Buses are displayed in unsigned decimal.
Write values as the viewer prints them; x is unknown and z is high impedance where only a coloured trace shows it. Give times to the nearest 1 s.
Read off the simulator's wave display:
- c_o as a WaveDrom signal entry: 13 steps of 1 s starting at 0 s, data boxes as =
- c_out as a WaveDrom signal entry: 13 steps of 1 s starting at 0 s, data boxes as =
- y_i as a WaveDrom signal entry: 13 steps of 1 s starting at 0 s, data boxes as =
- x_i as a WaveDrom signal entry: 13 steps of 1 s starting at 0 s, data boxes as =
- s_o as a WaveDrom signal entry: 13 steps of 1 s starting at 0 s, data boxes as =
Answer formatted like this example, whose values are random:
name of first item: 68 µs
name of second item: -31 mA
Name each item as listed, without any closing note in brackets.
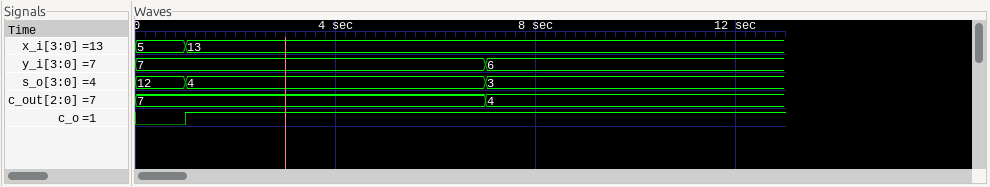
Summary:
c_o as a WaveDrom signal entry: 13 steps of 1 s starting at 0 s, data boxes as =: {name: 'c_o', wave: '01...........'}
c_out as a WaveDrom signal entry: 13 steps of 1 s starting at 0 s, data boxes as =: {name: 'c_out', wave: '=......=.....', data: '7 4'}
y_i as a WaveDrom signal entry: 13 steps of 1 s starting at 0 s, data boxes as =: {name: 'y_i', wave: '=......=.....', data: '7 6'}
x_i as a WaveDrom signal entry: 13 steps of 1 s starting at 0 s, data boxes as =: {name: 'x_i', wave: '==...........', data: '5 13'}
s_o as a WaveDrom signal entry: 13 steps of 1 s starting at 0 s, data boxes as =: {name: 's_o', wave: '==.....=.....', data: '12 4 3'}
